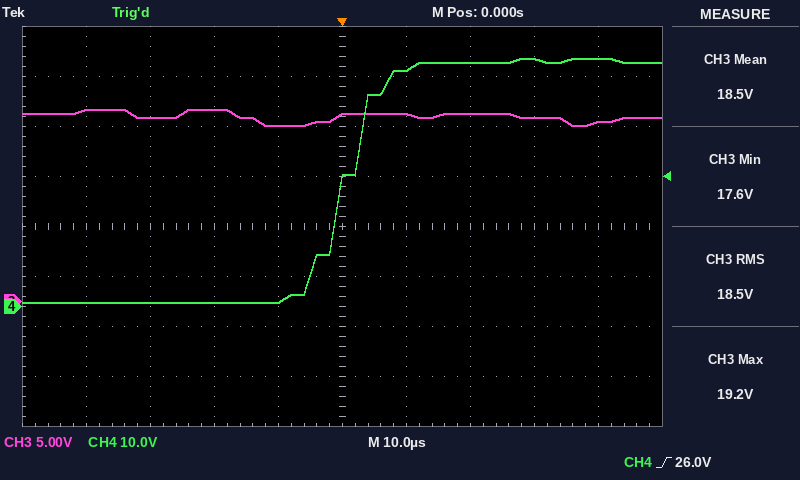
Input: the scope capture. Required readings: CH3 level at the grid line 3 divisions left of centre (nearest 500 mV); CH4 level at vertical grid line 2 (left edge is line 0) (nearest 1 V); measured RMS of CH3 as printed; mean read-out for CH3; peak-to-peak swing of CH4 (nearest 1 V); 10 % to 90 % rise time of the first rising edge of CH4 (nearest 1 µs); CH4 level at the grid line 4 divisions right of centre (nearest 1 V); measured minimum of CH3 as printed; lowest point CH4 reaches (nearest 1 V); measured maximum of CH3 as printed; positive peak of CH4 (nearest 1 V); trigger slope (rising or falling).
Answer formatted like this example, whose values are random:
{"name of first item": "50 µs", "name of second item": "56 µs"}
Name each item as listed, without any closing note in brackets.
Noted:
{"CH3 level at the grid line 3 divisions left of centre": "18.5 V", "CH4 level at vertical grid line 2 (left edge is line 0)": "1 V", "measured RMS of CH3 as printed": "18.5 V", "mean read-out for CH3": "18.5 V", "peak-to-peak swing of CH4": "49 V", "10 % to 90 % rise time of the first rising edge of CH4": "12 µs", "CH4 level at the grid line 4 divisions right of centre": "50 V", "measured minimum of CH3 as printed": "17.6 V", "lowest point CH4 reaches": "1 V", "measured maximum of CH3 as printed": "19.2 V", "positive peak of CH4": "50 V", "trigger slope": "rising"}
